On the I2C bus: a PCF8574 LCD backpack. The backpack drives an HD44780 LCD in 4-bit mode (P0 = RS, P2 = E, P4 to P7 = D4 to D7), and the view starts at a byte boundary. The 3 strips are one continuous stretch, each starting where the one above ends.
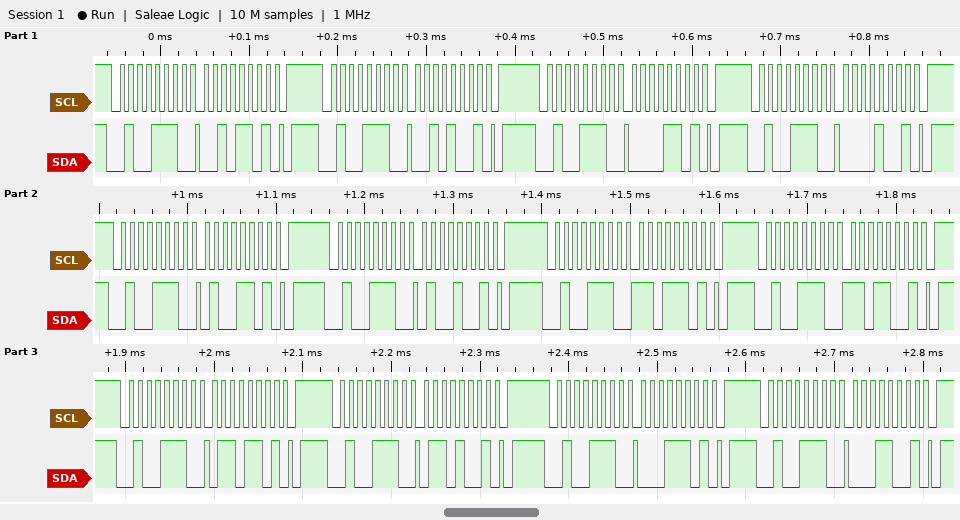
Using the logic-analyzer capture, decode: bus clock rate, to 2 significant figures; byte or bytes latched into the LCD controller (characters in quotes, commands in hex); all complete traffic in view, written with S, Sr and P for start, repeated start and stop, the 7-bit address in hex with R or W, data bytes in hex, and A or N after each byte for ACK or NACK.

100 kHz
' ' 'M' 'a'
S 27W A 2D A P S 27W A 29 A P S 27W A 0D A P S 27W A 09 A P S 27W A 4D A P S 27W A 49 A P S 27W A DD A P S 27W A D9 A P S 27W A 6D A P S 27W A 69 A P S 27W A 1D A P S 27W A 19 A P
